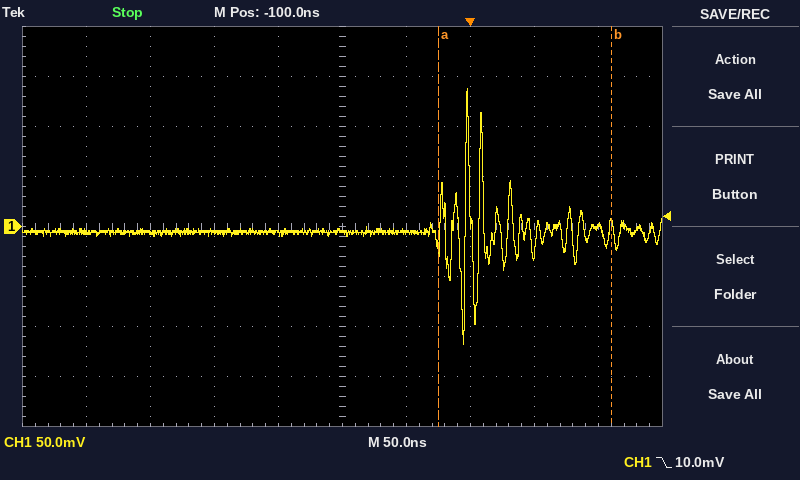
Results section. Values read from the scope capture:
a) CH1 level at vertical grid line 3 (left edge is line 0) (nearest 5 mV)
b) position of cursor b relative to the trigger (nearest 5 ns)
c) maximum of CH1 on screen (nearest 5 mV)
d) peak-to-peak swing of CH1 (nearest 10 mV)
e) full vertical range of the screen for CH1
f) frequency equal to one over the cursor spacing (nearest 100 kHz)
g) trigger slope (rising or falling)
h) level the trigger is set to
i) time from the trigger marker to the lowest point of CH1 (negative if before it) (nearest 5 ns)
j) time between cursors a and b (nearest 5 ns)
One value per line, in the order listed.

-5 mV
+110 ns
140 mV
260 mV
400 mV
7.4 MHz
falling
10.0 mV
-5 ns
135 ns
